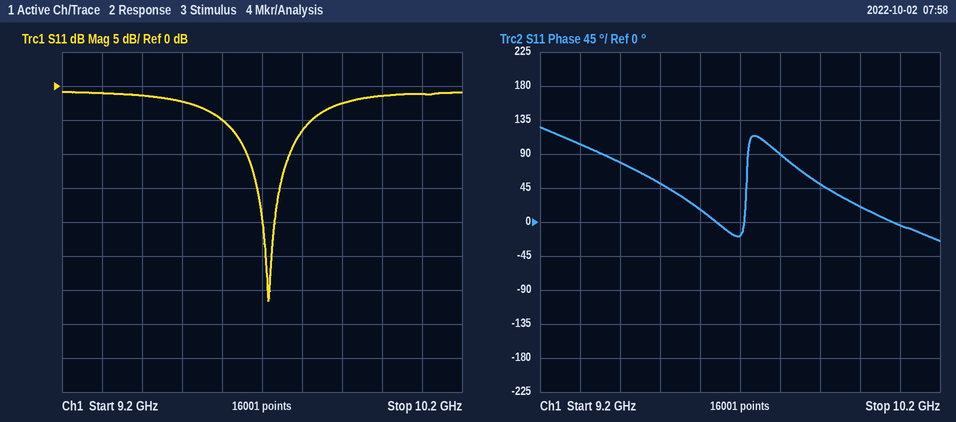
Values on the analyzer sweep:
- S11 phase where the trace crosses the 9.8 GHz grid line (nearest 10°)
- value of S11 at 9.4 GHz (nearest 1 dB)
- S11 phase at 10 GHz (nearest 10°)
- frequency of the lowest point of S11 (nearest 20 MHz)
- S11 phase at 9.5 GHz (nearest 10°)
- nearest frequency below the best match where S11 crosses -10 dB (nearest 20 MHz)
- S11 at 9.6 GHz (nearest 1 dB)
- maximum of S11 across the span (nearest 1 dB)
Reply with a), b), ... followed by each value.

a) 90°
b) -1 dB
c) 20°
d) 9.72 GHz
e) 50°
f) 9.66 GHz
g) -5 dB
h) -1 dB
